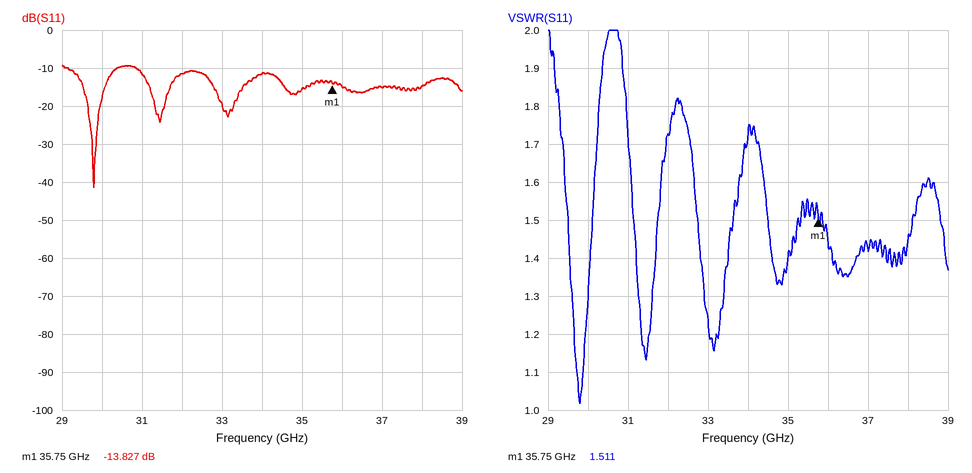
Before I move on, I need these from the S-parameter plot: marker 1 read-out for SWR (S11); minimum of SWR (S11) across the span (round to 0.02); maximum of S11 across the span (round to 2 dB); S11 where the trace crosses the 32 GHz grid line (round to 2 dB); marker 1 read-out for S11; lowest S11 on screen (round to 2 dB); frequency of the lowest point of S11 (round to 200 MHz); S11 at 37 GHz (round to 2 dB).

1.511
1.02
-10 dB
-12 dB
-13.827 dB
-42 dB
29.8 GHz
-16 dB
